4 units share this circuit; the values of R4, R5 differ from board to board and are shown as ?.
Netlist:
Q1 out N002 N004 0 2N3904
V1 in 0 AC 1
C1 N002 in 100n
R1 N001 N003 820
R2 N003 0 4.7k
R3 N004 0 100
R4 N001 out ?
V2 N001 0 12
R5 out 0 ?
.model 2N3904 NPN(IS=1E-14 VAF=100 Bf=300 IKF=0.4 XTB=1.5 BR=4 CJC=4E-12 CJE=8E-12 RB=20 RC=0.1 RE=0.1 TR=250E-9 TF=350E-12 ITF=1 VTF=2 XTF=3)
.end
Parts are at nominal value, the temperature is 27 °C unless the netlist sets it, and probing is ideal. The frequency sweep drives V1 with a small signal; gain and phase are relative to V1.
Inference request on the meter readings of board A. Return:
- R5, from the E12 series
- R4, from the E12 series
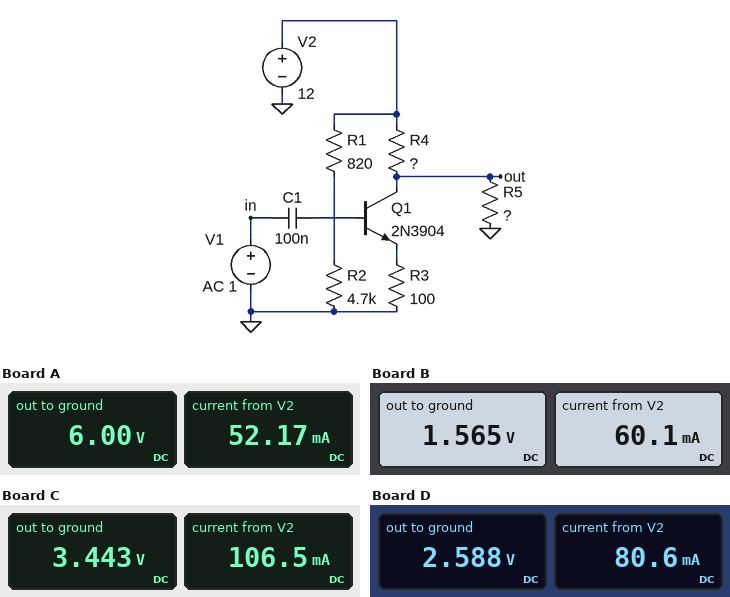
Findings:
120 Ω
120 Ω
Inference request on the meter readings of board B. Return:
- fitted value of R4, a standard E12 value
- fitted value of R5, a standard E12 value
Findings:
180 Ω
27 Ω
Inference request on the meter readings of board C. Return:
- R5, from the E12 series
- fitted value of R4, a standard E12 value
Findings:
33 Ω
82 Ω
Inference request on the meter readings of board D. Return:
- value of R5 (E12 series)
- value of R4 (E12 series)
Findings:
33 Ω
120 Ω
